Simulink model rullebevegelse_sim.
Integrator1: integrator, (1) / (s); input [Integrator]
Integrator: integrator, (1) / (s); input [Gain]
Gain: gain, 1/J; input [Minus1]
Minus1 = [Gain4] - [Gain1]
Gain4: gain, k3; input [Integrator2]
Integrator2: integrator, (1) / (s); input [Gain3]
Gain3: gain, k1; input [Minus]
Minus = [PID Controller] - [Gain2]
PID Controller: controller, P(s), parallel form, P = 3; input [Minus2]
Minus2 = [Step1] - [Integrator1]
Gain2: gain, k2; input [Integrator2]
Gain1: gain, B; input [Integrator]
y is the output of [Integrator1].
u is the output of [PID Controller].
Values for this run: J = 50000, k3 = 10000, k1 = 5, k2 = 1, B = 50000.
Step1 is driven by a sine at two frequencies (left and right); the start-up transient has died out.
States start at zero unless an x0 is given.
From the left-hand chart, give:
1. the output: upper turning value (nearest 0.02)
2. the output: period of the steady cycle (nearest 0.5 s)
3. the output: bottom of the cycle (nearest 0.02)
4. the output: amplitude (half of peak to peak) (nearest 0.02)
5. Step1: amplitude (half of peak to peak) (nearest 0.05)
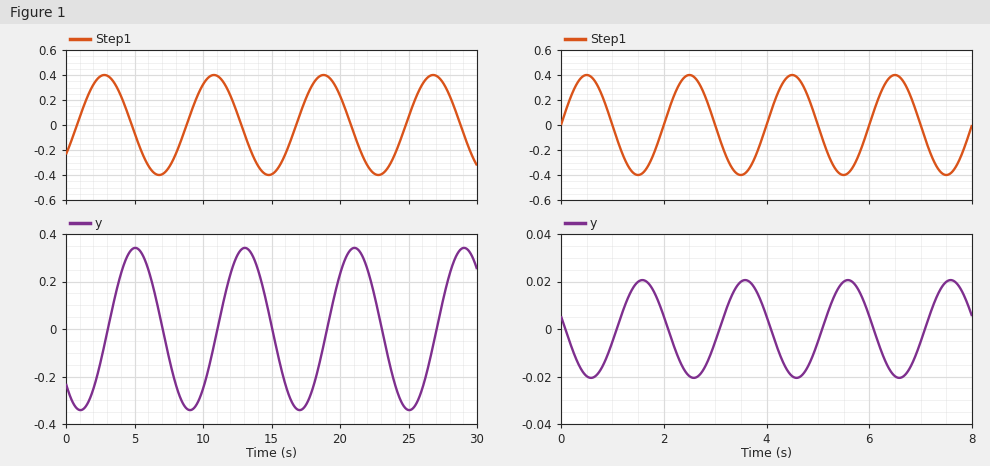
0.34
8.0 s
-0.34
0.34
0.40
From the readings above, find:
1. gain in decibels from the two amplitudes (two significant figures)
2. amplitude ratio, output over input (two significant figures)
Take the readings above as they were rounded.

-1.4 dB
0.85
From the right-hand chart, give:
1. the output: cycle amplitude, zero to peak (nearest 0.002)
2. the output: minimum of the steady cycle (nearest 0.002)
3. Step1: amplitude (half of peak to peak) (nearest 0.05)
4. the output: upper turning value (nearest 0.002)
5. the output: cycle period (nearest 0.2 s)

0.020
-0.020
0.40
0.020
2.0 s
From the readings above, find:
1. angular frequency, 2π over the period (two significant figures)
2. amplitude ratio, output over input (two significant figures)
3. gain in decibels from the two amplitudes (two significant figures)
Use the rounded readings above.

3.1 rad/s
0.050
-26 dB
